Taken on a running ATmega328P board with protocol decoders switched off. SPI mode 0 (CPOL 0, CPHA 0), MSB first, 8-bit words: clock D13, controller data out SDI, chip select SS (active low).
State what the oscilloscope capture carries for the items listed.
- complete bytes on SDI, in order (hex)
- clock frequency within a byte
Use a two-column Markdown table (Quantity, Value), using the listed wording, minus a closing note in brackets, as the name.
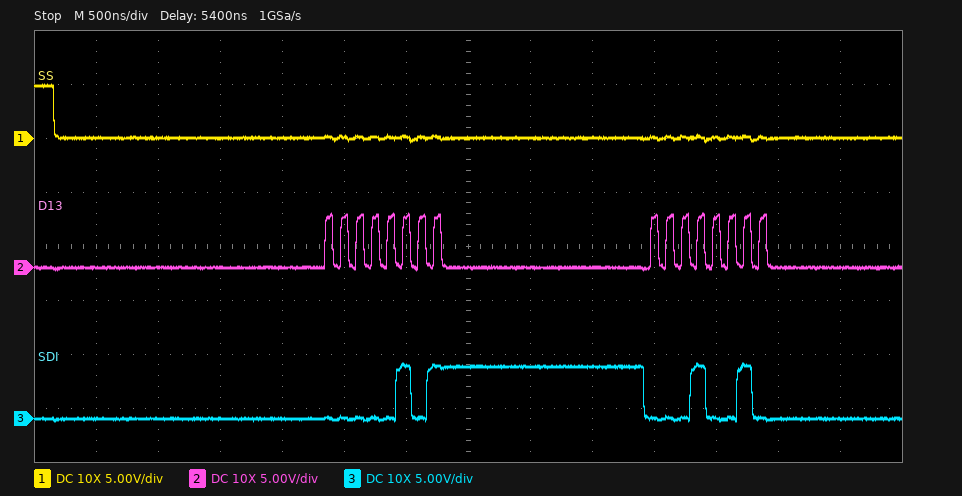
| Quantity | Value |
|---|---|
| complete bytes on SDI, in order | 0x05 0x12 |
| clock frequency within a byte | 8 MHz |
